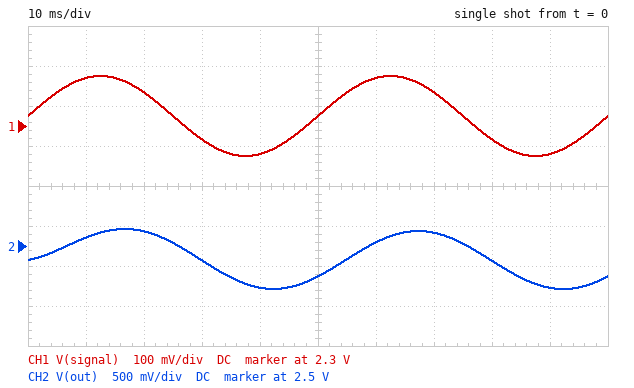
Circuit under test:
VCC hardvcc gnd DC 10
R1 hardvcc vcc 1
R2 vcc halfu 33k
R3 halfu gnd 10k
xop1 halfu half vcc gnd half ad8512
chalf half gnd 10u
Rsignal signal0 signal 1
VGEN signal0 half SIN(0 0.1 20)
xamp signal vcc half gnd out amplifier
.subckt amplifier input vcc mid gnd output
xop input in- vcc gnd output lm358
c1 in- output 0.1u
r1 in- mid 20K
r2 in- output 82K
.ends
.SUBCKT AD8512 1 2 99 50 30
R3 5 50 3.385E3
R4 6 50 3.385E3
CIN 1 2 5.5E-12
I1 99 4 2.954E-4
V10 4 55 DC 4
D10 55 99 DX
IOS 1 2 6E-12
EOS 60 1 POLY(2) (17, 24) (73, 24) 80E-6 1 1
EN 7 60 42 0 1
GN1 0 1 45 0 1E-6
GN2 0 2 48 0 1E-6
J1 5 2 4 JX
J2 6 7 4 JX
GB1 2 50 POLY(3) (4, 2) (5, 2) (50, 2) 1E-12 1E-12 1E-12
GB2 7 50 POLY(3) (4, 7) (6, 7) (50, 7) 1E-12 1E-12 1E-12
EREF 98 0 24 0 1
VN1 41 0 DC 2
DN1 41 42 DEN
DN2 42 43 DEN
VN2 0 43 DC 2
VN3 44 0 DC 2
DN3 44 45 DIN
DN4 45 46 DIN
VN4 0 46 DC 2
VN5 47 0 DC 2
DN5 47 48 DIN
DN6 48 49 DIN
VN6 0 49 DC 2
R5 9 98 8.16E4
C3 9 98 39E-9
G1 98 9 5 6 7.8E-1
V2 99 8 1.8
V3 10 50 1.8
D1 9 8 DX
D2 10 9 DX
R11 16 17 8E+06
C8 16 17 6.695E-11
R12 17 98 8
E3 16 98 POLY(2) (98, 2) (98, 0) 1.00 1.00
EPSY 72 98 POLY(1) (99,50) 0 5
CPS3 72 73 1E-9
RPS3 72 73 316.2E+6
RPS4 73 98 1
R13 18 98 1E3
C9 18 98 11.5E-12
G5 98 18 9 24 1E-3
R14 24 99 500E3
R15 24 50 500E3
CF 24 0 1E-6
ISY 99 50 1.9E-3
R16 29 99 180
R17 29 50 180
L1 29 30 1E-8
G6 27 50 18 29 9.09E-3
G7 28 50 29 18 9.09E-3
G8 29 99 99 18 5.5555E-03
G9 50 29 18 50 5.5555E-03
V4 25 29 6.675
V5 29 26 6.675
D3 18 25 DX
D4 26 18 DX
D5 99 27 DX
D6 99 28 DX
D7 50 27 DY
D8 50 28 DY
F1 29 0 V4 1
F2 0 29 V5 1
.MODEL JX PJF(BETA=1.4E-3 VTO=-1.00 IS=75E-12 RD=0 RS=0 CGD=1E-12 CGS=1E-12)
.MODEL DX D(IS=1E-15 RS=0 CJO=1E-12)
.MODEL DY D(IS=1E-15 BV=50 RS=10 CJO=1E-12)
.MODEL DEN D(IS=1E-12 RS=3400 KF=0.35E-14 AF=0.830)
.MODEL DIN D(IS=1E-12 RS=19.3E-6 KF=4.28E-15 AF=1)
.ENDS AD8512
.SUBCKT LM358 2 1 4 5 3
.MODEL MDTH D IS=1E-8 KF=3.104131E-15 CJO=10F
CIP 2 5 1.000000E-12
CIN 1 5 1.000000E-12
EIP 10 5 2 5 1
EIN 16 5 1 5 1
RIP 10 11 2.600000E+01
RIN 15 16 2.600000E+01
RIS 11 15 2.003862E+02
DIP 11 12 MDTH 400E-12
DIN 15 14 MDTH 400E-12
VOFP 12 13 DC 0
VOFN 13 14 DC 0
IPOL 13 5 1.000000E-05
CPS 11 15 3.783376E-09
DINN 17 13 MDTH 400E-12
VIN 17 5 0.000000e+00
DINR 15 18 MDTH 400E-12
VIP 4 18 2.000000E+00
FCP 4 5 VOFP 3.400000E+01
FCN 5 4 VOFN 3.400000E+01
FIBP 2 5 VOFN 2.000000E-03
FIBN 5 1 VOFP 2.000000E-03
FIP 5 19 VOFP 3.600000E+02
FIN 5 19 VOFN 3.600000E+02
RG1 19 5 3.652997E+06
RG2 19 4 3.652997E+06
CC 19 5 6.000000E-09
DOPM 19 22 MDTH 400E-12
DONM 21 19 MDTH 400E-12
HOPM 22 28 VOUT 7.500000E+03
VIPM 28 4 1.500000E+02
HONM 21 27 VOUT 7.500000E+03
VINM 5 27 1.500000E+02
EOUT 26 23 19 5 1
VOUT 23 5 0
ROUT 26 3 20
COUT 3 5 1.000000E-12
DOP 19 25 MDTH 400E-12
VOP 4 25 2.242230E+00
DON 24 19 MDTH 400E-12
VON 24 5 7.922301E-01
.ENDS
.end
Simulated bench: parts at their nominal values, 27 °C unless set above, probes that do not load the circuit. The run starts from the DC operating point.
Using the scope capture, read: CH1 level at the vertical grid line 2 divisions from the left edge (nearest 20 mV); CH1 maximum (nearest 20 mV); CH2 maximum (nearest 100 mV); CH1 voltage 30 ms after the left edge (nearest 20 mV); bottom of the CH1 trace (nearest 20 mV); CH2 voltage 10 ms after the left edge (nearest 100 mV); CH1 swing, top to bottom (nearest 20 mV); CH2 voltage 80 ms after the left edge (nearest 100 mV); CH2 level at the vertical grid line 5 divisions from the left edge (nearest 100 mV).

2.38 V
2.42 V
2.7 V
2.26 V
2.22 V
2.6 V
200 mV
2.3 V
2.1 V
